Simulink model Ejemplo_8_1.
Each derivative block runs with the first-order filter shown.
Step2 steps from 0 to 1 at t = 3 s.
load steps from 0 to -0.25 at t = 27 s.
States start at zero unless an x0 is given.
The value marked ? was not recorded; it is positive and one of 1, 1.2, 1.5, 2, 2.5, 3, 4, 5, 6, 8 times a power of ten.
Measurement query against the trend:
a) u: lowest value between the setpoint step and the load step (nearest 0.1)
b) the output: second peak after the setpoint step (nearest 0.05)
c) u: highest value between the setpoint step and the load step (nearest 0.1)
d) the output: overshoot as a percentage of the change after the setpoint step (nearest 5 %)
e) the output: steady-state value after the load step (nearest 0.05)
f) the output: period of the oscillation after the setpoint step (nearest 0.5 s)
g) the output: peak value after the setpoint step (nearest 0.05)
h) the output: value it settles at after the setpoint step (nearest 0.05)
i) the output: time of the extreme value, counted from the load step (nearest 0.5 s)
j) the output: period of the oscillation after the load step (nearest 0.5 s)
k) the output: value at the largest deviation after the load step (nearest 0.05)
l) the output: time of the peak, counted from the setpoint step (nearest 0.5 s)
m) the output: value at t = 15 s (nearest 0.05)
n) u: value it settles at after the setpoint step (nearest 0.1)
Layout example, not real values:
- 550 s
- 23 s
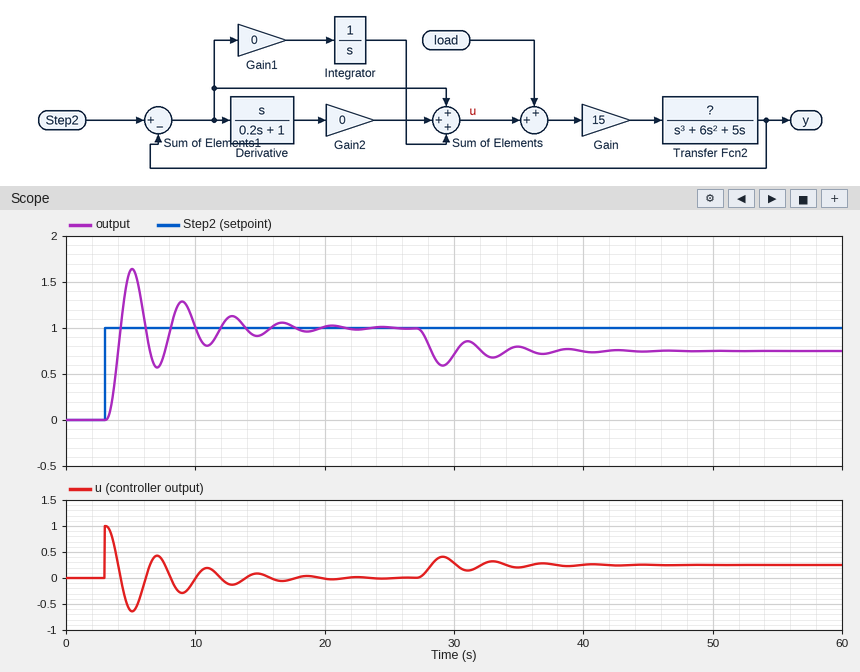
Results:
- -0.6
- 1.30
- 1.0
- 65 %
- 0.75
- 4.0 s
- 1.65
- 1.00
- 2.0 s
- 4.0 s
- 0.60
- 2.0 s
- 0.90
- 0.0
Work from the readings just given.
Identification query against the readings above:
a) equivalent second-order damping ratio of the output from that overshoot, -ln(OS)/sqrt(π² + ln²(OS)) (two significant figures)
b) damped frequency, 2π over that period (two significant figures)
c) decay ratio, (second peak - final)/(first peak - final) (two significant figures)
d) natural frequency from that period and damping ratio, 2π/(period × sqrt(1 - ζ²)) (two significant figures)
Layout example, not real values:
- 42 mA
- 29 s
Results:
- 0.14
- 1.6 rad/s
- 0.46
- 1.6 rad/s
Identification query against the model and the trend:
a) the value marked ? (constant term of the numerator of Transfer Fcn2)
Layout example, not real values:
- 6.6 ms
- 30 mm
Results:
- 1
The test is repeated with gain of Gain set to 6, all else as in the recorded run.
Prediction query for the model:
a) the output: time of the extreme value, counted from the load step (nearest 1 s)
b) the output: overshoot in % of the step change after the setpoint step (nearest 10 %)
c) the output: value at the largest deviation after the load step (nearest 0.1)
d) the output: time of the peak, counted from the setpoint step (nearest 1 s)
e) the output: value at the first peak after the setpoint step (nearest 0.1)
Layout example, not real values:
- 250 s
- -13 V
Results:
- 3 s
- 30 %
- 0.7
- 3 s
- 1.3
